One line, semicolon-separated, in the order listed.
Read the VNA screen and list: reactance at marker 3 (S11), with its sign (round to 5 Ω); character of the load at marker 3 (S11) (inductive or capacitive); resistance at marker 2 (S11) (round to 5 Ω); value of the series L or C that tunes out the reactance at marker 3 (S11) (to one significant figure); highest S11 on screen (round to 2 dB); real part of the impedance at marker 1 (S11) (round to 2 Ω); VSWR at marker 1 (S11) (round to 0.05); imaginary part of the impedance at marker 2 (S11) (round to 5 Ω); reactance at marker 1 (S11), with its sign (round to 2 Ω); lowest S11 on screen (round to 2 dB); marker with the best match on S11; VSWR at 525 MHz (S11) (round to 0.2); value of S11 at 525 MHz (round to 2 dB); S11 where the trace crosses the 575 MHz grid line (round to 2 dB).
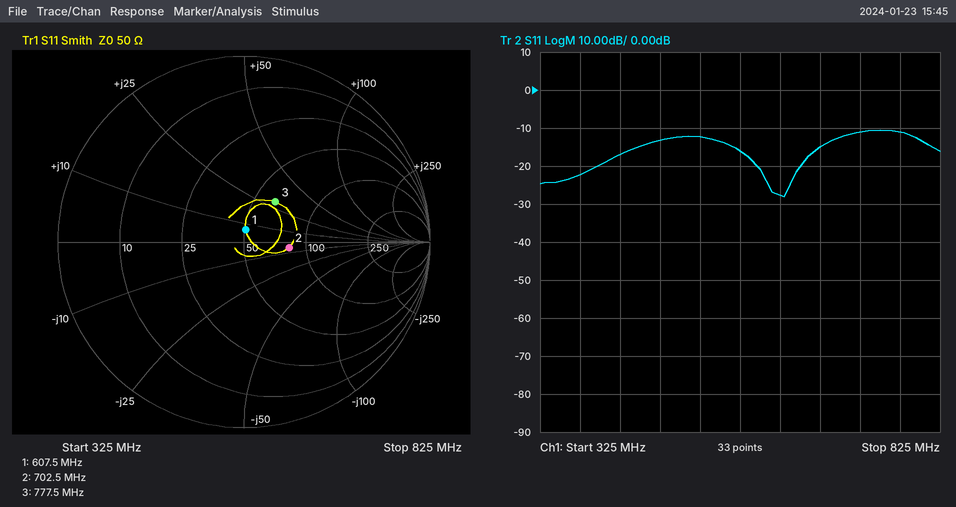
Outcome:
+30 Ω; inductive; 80 Ω; 7 pF; -10 dB; 50 Ω; 1.15; -5 Ω; +6 Ω; -28 dB; marker 1; 1.6; -12 dB; -16 dB
